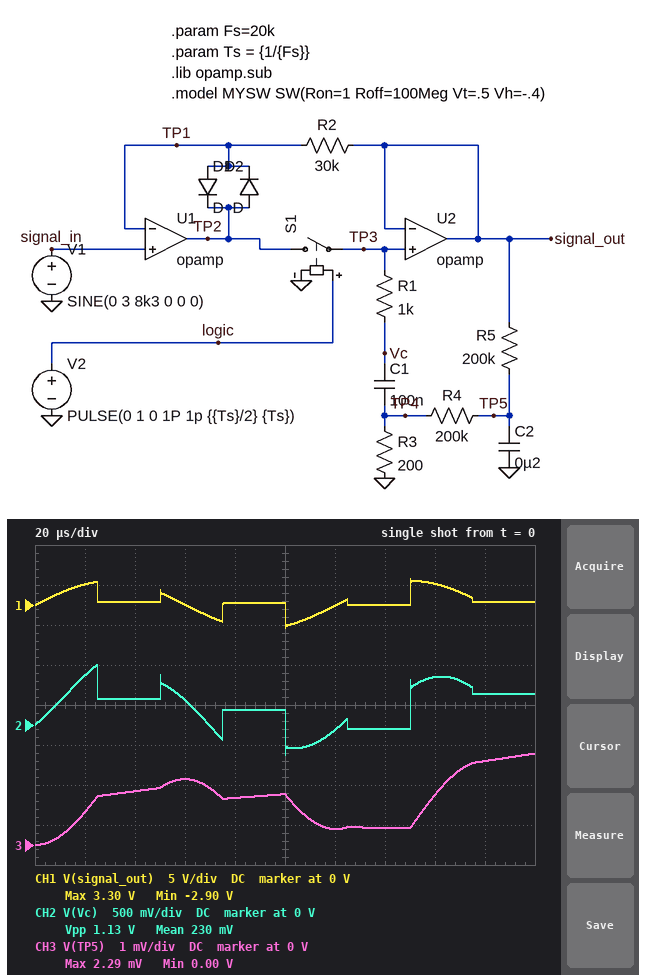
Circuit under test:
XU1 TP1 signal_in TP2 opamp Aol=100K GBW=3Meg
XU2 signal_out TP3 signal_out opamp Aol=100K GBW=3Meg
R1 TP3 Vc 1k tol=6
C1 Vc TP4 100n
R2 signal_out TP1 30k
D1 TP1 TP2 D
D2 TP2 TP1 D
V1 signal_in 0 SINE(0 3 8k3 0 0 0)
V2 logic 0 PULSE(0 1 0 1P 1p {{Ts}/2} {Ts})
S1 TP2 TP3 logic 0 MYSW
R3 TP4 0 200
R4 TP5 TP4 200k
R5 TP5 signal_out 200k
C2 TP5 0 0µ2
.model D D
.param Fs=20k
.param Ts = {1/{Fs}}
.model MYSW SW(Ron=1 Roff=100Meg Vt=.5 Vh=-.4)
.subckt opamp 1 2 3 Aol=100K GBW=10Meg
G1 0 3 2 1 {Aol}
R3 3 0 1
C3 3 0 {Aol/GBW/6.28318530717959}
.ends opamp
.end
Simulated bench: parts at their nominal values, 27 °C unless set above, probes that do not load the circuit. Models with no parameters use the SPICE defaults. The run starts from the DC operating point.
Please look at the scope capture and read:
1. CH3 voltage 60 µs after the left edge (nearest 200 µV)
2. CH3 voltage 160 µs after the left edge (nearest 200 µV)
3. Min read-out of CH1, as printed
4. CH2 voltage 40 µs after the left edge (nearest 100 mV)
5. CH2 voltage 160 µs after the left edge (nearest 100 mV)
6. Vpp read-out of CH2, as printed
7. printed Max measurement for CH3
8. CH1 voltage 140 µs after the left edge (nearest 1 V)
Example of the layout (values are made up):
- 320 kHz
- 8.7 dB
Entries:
- 1.6 mV
- 1.2 mV
- -2.90 V
- 300 mV
- 600 mV
- 1.13 V
- 2.29 mV
- 0 V
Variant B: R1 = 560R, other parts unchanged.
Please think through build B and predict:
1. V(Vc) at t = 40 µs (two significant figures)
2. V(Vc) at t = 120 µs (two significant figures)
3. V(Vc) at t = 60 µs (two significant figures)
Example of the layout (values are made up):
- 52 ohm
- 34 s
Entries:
- 500 mV
- -130 mV
- 400 mV
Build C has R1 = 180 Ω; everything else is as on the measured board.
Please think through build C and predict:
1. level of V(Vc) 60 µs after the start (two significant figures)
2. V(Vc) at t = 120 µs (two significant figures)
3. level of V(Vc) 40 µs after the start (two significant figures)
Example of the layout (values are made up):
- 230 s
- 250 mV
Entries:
- 430 mV
- -250 mV
- 890 mV
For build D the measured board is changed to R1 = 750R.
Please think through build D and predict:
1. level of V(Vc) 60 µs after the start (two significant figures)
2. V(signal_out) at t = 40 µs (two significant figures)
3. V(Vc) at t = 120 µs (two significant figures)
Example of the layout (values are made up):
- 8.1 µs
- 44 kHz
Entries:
- 360 mV
- 410 mV
- -93 mV
